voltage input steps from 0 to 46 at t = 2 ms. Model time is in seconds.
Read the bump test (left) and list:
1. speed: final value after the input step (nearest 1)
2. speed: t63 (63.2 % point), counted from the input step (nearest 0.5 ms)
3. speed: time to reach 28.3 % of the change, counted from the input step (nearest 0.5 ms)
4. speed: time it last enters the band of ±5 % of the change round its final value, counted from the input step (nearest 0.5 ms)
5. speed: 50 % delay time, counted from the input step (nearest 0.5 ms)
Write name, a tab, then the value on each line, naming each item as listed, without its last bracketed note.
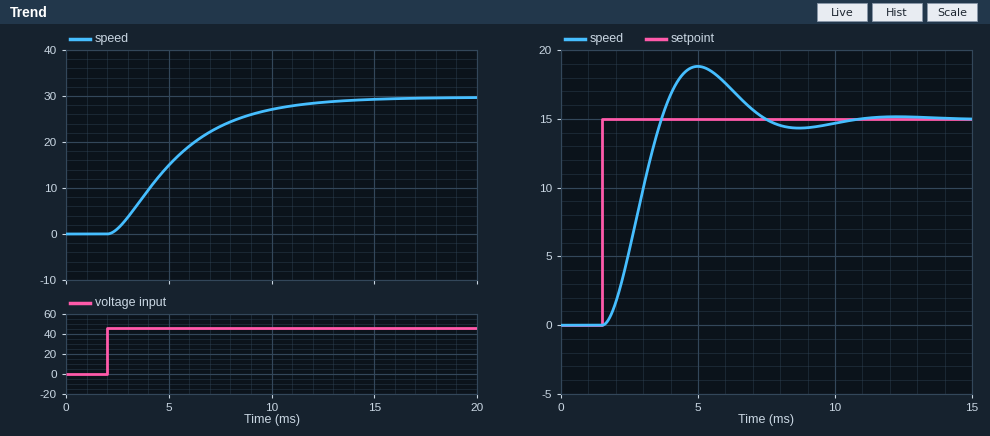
speed: final value after the input step	30
speed: t63 (63.2 % point), counted from the input step	4.0 ms
speed: time to reach 28.3 % of the change, counted from the input step	2.0 ms
speed: time it last enters the band of ±5 % of the change round its final value, counted from the input step	9.5 ms
speed: 50 % delay time, counted from the input step	3.0 ms
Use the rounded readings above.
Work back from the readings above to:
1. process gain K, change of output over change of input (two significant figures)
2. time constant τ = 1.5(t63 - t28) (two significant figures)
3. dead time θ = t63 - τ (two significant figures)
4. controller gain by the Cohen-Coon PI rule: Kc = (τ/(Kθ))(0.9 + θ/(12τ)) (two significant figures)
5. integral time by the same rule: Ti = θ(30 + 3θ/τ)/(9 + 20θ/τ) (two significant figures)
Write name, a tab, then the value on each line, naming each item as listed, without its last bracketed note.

process gain K, change of output over change of input	0.65
time constant τ = 1.5(t63 - t28)	3.0 ms
dead time θ = t63 - τ	1.0 ms
controller gain by the Cohen-Coon PI rule: Kc = (τ/(Kθ))(0.9 + θ/(12τ))	4.3
integral time by the same rule: Ti = θ(30 + 3θ/τ)/(9 + 20θ/τ)	2.0 ms
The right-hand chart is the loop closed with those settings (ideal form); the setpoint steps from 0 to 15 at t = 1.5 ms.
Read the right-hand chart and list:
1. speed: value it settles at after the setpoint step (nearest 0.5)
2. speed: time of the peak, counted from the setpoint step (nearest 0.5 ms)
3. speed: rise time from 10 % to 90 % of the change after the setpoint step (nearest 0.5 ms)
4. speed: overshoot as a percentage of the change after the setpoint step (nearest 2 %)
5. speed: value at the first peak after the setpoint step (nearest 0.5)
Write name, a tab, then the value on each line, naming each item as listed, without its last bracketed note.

speed: value it settles at after the setpoint step	15.0
speed: time of the peak, counted from the setpoint step	3.5 ms
speed: rise time from 10 % to 90 % of the change after the setpoint step	1.5 ms
speed: overshoot as a percentage of the change after the setpoint step	26 %
speed: value at the first peak after the setpoint step	19.0
